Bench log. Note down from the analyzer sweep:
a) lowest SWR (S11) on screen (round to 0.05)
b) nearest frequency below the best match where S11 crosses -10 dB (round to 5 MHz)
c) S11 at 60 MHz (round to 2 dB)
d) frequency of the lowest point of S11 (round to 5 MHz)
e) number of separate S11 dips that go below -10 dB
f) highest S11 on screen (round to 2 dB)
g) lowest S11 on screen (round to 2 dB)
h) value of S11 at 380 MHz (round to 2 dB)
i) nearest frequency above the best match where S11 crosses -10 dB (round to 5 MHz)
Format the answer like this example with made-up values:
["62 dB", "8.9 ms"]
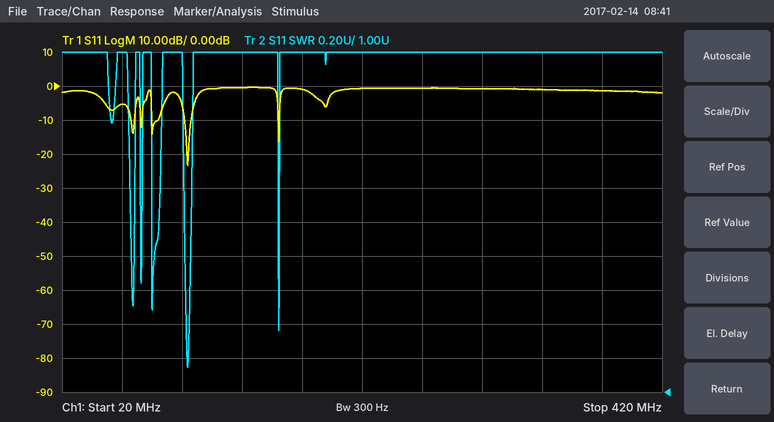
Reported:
["1.15", "100 MHz", "-6 dB", "105 MHz", "5", "0 dB", "-24 dB", "-2 dB", "105 MHz"]
